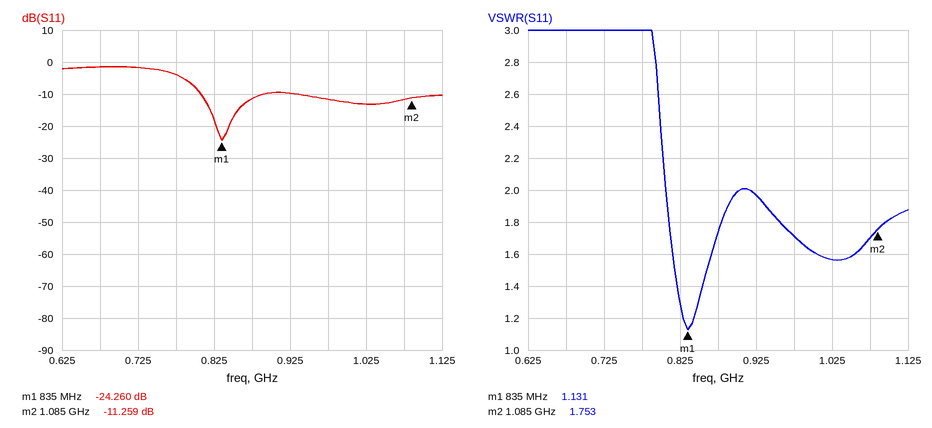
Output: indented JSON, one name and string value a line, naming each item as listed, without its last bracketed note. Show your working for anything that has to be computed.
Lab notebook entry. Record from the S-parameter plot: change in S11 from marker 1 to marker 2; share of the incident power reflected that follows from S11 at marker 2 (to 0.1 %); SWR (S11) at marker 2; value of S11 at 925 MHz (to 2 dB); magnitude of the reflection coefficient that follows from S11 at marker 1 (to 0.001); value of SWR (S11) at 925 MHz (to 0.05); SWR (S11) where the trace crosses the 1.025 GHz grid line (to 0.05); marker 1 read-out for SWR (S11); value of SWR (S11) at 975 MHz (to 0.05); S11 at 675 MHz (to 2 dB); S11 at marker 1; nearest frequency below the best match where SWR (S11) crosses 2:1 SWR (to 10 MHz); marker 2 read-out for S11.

{
  "change in S11 from marker 1 to marker 2": "-11.259 − (-24.26) = 13.001 dB",
  "share of the incident power reflected that follows from S11 at marker 2": "10^(-11.259/10) ≈ 7.5 %",
  "SWR (S11) at marker 2": "1.753",
  "value of S11 at 925 MHz": "-10 dB",
  "magnitude of the reflection coefficient that follows from S11 at marker 1": "10^(-24.26/20) ≈ 0.061",
  "value of SWR (S11) at 925 MHz": "1.95",
  "SWR (S11) where the trace crosses the 1.025 GHz grid line": "1.55",
  "marker 1 read-out for SWR": "1.131",
  "value of SWR (S11) at 975 MHz": "1.70",
  "S11 at 675 MHz": "-2 dB",
  "S11 at marker 1": "-24.260 dB",
  "nearest frequency below the best match where SWR (S11) crosses 2:1 SWR": "810 MHz",
  "marker 2 read-out for S11": "-11.259 dB"
}
